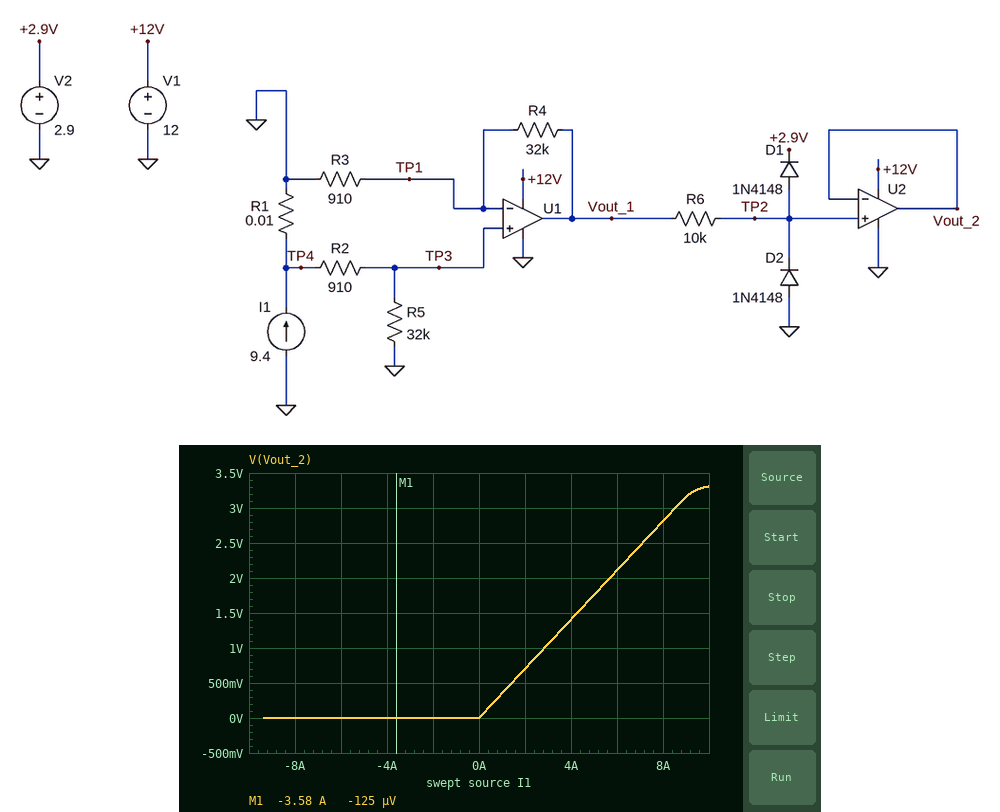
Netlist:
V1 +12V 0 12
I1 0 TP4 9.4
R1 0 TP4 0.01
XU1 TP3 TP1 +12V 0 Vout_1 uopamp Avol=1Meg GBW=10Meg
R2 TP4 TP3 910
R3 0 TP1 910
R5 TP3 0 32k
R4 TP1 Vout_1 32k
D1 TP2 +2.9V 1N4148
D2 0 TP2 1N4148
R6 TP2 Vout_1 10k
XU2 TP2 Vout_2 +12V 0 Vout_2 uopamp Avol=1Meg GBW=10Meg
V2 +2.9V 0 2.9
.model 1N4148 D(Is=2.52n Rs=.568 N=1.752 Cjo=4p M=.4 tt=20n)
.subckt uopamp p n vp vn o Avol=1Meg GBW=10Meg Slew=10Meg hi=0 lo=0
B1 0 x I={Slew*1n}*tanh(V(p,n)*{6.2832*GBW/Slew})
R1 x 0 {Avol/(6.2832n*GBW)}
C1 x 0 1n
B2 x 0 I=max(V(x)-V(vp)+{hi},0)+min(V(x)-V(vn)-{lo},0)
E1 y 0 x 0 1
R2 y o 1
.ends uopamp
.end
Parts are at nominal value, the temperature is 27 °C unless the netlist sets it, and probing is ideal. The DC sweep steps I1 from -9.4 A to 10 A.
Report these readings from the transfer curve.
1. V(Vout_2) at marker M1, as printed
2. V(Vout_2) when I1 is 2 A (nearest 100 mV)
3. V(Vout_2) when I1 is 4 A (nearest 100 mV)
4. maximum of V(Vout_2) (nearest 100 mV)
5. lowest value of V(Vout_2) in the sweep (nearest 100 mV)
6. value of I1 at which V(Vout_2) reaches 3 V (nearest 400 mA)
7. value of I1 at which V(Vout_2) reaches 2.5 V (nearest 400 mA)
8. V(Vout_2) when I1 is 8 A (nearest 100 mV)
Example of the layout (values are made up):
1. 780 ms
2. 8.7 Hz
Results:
1. -125 µV
2. 700 mV
3. 1.4 V
4. 3.3 V
5. 0 V
6. 8.4 A
7. 7.2 A
8. 2.8 V
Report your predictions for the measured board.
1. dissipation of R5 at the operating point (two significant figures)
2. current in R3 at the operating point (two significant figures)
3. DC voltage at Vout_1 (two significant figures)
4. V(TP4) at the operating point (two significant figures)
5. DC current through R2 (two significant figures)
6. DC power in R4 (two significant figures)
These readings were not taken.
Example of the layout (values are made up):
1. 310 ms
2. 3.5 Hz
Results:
1. 260 nW
2. 100 µA
3. 3.3 V
4. 94 mV
5. 2.9 µA
6. 320 µW
